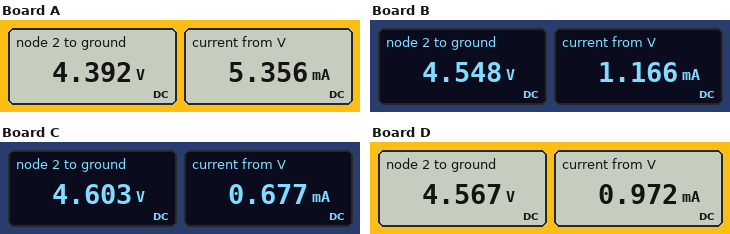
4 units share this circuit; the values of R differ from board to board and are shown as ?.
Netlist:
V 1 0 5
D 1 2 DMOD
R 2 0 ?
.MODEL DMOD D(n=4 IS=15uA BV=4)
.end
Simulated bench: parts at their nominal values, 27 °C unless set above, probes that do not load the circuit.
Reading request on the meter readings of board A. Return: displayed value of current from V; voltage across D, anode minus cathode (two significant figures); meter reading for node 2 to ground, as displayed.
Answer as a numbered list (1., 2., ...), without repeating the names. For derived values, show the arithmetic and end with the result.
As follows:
1. 5.356 mA
2. 5 V - 4.392 V = 610 mV
3. 4.392 V
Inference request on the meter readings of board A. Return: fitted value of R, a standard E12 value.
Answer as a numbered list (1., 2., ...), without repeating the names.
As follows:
1. 820 Ω
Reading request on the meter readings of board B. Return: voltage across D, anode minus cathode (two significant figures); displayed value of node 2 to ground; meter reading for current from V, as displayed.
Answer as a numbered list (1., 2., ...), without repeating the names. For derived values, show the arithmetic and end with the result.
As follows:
1. 5 V - 4.548 V = 450 mV
2. 4.548 V
3. 1.166 mA
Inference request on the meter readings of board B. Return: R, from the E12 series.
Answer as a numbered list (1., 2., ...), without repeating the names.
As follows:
1. 3.9 kΩ
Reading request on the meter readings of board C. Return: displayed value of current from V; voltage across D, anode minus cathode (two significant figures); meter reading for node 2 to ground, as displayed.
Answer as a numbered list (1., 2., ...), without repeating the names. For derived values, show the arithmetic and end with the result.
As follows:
1. 0.677 mA
2. 5 V - 4.603 V = 400 mV
3. 4.603 V
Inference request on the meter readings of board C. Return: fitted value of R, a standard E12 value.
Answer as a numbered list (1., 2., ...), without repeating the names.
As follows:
1. 6.8 kΩ
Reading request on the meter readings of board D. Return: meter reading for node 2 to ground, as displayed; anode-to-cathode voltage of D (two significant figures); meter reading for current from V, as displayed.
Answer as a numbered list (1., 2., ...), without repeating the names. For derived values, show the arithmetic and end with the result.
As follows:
1. 4.567 V
2. 5 V - 4.567 V = 430 mV
3. 0.972 mA
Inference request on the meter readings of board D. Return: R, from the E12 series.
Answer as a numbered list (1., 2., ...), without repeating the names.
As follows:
1. 4.7 kΩ
